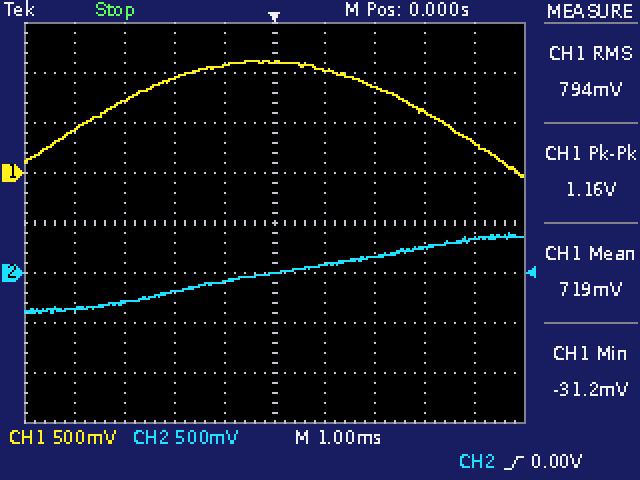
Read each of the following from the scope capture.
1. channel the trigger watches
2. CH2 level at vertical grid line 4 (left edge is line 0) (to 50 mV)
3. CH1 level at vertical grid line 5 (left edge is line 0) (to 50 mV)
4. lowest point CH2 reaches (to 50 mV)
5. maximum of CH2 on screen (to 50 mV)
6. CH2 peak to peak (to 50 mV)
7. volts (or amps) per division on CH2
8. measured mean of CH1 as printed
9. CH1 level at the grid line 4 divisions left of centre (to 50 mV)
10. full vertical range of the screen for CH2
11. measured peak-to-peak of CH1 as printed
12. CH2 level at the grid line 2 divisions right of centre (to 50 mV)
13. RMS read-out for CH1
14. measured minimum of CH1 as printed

CH2
-100 mV
1.10 V
-400 mV
400 mV
800 mV
500 mV
719 mV
450 mV
4 V
1.16 V
150 mV
794 mV
-31.2 mV
